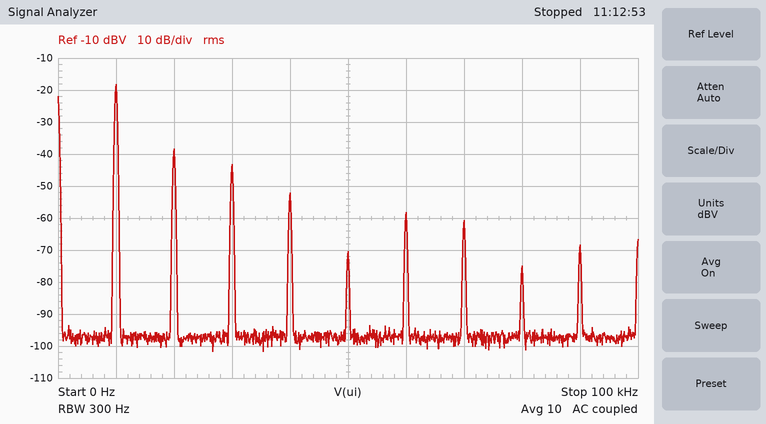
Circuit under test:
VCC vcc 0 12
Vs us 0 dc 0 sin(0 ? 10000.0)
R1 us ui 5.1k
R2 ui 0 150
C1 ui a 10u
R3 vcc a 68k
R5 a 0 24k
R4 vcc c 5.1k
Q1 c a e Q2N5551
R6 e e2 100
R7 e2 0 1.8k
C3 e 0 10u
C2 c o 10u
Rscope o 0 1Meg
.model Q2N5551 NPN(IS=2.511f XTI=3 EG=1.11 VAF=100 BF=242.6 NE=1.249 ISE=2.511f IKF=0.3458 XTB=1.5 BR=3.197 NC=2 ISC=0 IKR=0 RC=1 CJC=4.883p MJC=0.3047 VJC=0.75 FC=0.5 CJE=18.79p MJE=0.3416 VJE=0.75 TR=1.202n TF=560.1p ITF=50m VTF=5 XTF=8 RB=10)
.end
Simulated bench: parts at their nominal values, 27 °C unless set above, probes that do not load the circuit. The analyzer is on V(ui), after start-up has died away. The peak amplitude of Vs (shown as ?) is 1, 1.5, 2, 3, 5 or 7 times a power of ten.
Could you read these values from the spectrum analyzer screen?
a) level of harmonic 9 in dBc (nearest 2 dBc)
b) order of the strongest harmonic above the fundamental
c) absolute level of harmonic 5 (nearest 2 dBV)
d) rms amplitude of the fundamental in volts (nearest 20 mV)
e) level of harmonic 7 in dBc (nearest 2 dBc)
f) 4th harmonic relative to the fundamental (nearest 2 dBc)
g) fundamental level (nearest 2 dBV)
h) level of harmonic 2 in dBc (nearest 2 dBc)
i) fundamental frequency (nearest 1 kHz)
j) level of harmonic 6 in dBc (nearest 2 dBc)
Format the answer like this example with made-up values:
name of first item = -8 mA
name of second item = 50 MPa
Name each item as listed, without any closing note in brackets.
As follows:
level of harmonic 9 in dBc = -50 dBc
order of the strongest harmonic above the fundamental = 2
absolute level of harmonic 5 = -70 dBV
rms amplitude of the fundamental in volts = 120 mV
level of harmonic 7 in dBc = -42 dBc
4th harmonic relative to the fundamental = -34 dBc
fundamental level = -18 dBV
level of harmonic 2 in dBc = -20 dBc
fundamental frequency = 10 kHz
level of harmonic 6 in dBc = -40 dBc
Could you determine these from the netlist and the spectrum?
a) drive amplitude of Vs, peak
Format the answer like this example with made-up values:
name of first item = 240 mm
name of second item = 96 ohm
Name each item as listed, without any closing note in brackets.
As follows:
drive amplitude of Vs, peak = 7 V
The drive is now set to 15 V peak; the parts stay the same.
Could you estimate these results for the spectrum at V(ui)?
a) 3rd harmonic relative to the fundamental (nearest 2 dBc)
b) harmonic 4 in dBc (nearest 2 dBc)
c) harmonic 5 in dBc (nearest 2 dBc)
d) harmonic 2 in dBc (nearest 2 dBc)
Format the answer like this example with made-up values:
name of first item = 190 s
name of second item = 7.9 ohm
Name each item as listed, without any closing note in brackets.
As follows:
3rd harmonic relative to the fundamental = -26 dBc
harmonic 4 in dBc = -32 dBc
harmonic 5 in dBc = -42 dBc
harmonic 2 in dBc = -24 dBc
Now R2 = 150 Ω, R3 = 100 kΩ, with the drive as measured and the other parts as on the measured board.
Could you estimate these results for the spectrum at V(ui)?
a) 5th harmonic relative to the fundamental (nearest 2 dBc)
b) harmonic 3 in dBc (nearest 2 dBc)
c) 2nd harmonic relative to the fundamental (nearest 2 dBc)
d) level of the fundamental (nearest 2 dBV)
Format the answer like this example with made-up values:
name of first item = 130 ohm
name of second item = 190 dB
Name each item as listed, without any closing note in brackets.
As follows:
5th harmonic relative to the fundamental = -40 dBc
harmonic 3 in dBc = -28 dBc
2nd harmonic relative to the fundamental = -26 dBc
level of the fundamental = -18 dBV
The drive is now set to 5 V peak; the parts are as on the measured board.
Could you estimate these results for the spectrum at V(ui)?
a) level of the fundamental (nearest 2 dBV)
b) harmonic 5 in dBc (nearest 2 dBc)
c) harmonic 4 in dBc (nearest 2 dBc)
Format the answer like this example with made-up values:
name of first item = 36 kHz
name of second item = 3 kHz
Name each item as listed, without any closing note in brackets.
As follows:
level of the fundamental = -22 dBV
harmonic 5 in dBc = -42 dBc
harmonic 4 in dBc = -36 dBc
